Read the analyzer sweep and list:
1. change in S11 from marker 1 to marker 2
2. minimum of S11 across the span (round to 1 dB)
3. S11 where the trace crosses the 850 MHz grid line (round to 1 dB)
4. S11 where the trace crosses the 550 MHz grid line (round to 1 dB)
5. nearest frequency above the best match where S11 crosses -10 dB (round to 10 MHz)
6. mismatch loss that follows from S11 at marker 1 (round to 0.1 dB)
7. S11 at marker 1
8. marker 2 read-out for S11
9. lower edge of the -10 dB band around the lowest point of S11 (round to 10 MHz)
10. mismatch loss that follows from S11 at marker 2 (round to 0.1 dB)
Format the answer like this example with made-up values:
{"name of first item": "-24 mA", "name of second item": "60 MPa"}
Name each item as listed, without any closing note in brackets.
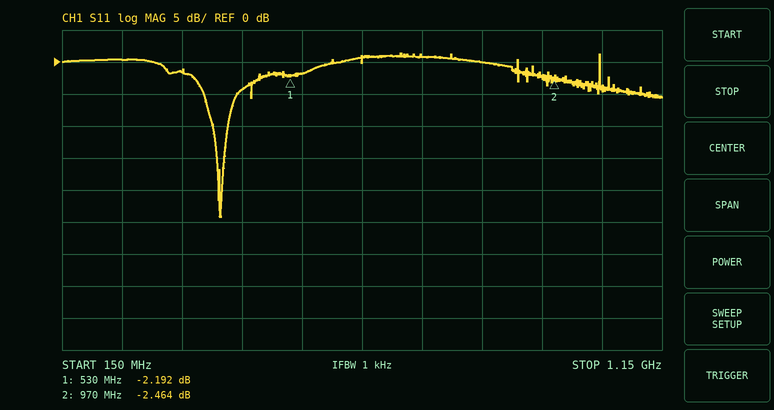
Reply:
{"change in S11 from marker 1 to marker 2": "-0.272 dB", "minimum of S11 across the span": "-24 dB", "S11 where the trace crosses the 850 MHz grid line": "0 dB", "S11 where the trace crosses the 550 MHz grid line": "-2 dB", "nearest frequency above the best match where S11 crosses -10 dB": "430 MHz", "mismatch loss that follows from S11 at marker 1": "4.0 dB", "S11 at marker 1": "-2.192 dB", "marker 2 read-out for S11": "-2.464 dB", "lower edge of the -10 dB band around the lowest point of S11": "400 MHz", "mismatch loss that follows from S11 at marker 2": "3.6 dB"}
